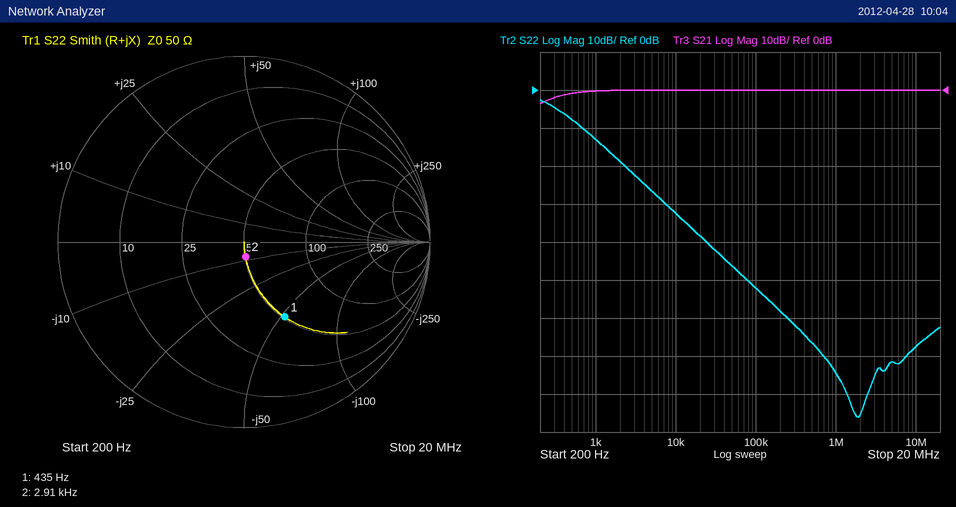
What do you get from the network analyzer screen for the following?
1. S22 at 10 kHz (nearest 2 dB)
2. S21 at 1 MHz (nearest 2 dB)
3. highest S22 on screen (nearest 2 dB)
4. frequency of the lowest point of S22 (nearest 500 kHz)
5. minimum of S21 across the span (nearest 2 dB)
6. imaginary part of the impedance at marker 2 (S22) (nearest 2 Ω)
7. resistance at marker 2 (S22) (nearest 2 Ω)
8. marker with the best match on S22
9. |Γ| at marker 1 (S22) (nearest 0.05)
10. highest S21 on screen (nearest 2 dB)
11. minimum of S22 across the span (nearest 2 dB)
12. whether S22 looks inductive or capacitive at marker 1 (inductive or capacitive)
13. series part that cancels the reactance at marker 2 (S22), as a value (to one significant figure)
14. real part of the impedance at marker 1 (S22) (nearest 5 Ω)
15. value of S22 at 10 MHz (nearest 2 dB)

-32 dB
0 dB
-2 dB
2.0 MHz
-4 dB
-8 Ω
50 Ω
marker 2
0.45
0 dB
-86 dB
capacitive
400 µH
50 Ω
-68 dB
